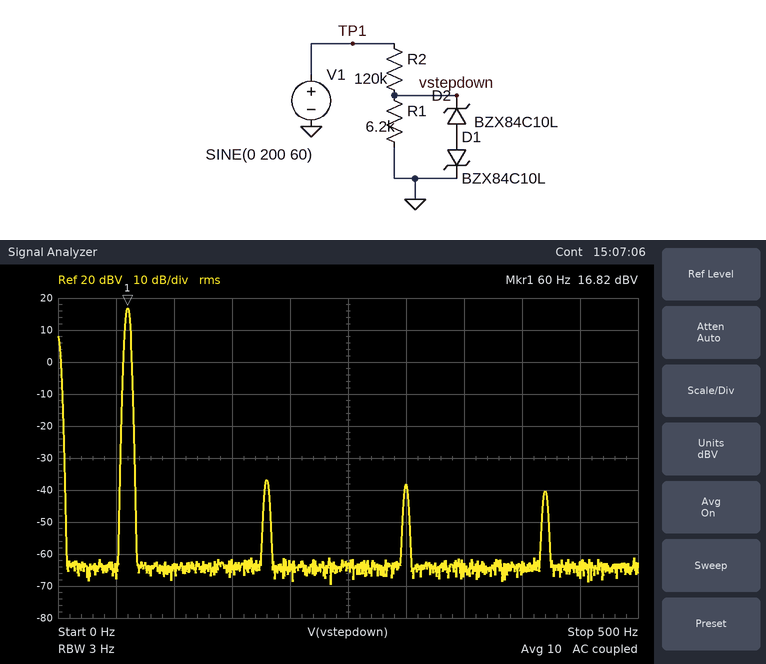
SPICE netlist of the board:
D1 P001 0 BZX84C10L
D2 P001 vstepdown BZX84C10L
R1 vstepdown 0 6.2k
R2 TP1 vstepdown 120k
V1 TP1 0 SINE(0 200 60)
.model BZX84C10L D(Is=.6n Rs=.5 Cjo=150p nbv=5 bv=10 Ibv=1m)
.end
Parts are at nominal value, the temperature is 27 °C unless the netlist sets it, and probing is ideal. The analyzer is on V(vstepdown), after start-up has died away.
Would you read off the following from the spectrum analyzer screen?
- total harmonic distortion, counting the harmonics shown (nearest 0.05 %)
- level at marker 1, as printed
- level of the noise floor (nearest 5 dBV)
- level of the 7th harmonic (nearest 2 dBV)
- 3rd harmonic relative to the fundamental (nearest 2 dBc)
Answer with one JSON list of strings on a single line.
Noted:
["0.30 %", "16.82 dBV", "-65 dBV", "-40 dBV", "-54 dBc"]
